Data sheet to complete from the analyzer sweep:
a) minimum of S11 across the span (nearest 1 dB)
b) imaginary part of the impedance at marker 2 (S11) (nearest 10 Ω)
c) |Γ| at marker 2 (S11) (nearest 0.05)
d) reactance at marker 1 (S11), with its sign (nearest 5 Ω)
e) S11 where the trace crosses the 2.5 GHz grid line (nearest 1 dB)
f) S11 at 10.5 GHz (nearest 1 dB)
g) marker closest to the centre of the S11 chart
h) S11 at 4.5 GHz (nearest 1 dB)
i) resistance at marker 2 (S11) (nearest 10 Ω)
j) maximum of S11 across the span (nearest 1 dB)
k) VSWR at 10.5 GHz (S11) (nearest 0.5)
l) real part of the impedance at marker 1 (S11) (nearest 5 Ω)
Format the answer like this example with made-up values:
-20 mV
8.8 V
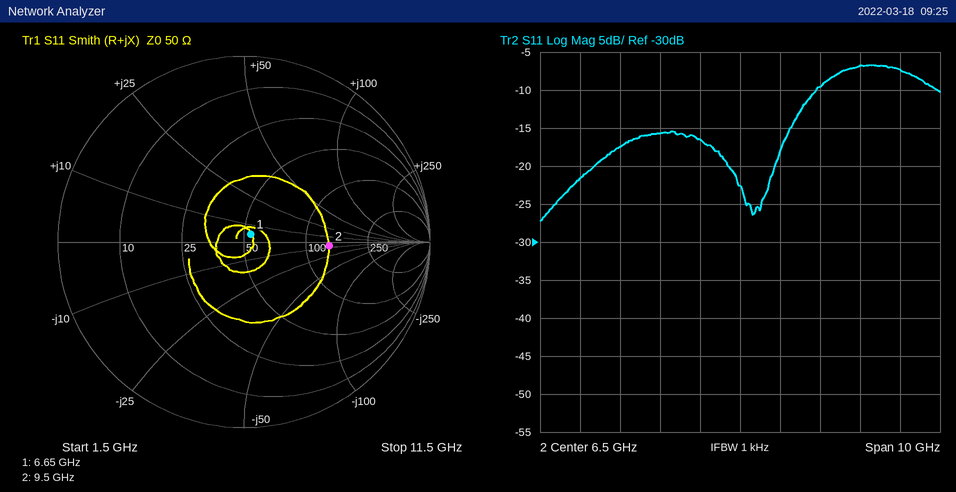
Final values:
-27 dB
-10 Ω
0.45
+5 Ω
-22 dB
-7 dB
marker 1
-16 dB
130 Ω
-7 dB
2.5
55 Ω
